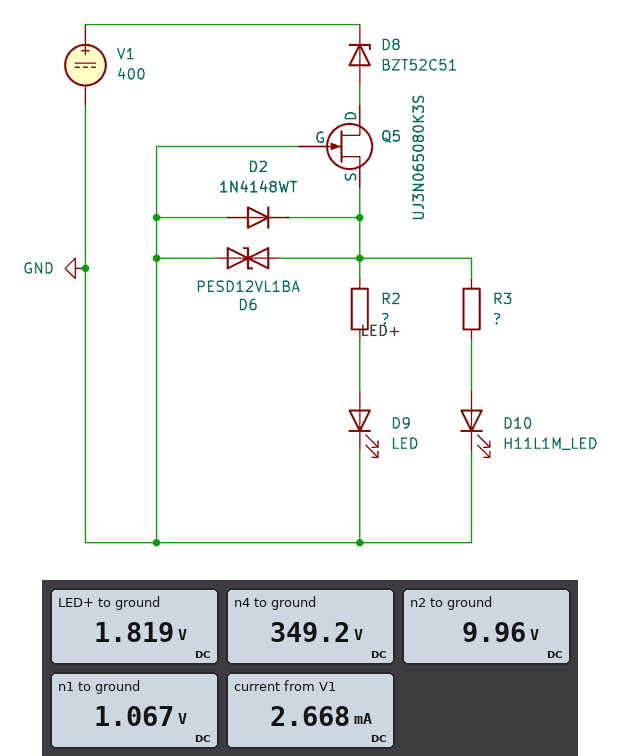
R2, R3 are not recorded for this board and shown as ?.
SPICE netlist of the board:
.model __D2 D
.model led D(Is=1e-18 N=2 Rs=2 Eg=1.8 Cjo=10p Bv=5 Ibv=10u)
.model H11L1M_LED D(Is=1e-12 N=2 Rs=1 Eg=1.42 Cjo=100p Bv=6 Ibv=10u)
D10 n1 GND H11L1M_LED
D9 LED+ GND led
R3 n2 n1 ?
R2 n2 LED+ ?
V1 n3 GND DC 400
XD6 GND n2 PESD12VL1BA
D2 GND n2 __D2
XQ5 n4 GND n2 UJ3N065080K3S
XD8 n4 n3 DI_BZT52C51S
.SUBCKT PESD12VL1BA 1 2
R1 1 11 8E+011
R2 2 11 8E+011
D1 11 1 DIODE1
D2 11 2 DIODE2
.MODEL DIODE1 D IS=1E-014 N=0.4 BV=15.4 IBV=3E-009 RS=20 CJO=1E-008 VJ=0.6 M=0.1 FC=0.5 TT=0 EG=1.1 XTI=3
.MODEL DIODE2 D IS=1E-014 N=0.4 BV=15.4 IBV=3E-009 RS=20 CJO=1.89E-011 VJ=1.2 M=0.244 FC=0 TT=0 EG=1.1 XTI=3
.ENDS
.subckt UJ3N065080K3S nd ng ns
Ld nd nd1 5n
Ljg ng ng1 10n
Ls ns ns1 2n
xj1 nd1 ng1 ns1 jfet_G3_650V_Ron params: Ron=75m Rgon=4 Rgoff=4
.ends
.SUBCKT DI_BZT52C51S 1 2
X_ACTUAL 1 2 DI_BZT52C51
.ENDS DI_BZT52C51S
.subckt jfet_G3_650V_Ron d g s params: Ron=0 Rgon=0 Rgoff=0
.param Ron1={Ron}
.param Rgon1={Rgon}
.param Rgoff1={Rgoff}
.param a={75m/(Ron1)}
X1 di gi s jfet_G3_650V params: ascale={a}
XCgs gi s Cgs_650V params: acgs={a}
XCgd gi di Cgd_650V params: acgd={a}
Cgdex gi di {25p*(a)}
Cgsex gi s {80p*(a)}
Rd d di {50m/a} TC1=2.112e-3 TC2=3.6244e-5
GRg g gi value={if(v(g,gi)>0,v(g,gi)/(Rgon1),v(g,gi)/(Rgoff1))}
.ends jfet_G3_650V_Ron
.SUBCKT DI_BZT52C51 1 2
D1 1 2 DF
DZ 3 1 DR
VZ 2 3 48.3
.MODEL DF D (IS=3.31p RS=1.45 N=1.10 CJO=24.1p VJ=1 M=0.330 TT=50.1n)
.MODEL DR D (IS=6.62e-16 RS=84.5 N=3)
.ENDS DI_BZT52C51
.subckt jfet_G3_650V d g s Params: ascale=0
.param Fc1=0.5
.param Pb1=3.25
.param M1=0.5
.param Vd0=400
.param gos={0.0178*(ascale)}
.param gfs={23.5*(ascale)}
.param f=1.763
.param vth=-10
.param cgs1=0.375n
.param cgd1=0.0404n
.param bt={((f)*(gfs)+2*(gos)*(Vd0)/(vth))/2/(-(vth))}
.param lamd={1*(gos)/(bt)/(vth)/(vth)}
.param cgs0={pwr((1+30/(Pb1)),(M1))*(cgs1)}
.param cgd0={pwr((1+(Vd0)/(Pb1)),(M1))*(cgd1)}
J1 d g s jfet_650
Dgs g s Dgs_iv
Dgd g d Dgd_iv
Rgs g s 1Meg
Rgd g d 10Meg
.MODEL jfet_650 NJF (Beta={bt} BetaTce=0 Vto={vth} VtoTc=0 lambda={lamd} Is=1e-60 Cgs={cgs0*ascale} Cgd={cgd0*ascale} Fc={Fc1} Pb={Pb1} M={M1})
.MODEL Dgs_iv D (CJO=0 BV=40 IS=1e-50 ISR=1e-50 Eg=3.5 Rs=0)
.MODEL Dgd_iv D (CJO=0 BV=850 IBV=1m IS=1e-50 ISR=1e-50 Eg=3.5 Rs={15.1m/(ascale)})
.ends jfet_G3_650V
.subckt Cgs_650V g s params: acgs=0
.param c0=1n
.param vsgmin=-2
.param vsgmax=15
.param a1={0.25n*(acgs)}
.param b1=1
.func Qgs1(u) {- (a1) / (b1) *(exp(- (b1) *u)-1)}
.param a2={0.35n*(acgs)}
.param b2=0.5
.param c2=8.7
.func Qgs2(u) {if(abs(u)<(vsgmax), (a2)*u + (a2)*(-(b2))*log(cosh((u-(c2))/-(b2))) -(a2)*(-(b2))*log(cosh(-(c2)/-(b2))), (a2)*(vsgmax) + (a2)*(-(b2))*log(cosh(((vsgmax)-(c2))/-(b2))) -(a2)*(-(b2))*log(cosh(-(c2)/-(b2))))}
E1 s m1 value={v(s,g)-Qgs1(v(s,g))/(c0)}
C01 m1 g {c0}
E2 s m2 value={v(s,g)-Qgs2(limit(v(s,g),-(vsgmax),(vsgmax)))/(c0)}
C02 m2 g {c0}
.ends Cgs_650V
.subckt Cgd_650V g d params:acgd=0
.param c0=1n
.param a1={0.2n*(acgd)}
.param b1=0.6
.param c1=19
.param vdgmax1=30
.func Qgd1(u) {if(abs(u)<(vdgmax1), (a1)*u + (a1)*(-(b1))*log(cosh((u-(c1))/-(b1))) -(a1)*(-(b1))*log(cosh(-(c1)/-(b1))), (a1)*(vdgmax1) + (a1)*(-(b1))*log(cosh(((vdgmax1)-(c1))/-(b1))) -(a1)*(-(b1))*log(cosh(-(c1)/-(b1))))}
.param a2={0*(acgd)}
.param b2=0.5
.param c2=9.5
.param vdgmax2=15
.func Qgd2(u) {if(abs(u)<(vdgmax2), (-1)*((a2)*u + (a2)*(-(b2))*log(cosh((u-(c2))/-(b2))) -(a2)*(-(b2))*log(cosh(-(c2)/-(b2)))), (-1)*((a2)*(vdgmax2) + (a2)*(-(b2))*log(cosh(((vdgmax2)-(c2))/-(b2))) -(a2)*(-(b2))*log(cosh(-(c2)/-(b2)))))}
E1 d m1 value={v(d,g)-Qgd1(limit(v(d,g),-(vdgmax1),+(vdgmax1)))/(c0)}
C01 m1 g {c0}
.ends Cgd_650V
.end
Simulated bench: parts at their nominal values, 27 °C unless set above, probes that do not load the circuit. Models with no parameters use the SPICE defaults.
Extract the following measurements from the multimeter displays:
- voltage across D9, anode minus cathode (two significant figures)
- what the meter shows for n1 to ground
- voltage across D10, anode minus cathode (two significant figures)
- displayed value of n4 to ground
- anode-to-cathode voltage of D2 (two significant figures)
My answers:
1.8 V
1.067 V
1.1 V
349.2 V
-10 V
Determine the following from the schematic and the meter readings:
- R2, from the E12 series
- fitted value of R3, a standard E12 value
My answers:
4.7 kΩ
10 kΩ
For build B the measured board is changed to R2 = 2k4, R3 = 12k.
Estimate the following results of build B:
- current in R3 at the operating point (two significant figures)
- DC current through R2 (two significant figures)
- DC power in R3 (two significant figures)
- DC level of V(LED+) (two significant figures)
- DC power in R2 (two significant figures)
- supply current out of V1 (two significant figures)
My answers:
740 µA
3.4 mA
6.6 mW
1.9 V
27 mW
4.2 mA
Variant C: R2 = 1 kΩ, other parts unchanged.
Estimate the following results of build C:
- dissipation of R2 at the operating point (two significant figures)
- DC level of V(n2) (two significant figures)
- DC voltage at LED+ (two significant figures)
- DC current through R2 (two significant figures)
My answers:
64 mW
9.9 V
1.9 V
8.0 mA
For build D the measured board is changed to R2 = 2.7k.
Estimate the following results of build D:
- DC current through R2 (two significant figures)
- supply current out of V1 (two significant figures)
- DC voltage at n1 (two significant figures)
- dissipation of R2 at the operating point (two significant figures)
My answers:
3.0 mA
3.9 mA
1.1 V
24 mW
